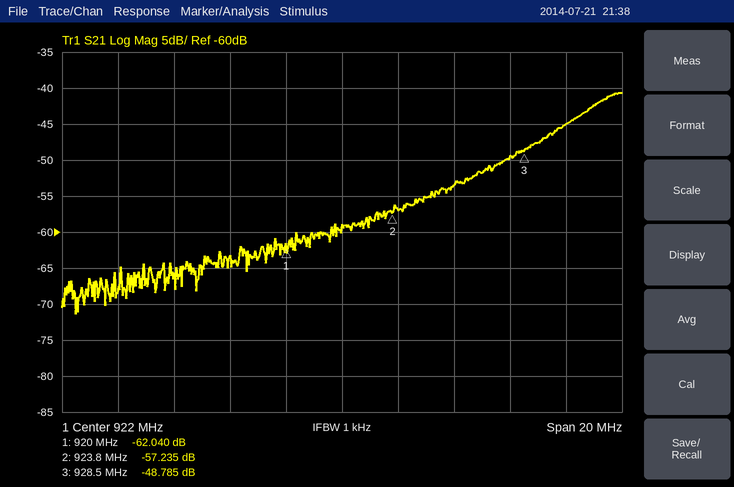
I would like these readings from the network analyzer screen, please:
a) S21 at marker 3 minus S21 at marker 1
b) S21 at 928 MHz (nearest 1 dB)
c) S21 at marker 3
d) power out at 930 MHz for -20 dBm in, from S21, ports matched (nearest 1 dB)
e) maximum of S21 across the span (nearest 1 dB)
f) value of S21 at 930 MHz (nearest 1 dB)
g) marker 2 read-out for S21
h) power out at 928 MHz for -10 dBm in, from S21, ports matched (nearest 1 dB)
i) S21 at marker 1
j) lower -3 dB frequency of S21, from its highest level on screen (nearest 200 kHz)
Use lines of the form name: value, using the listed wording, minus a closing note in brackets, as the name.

S21 at marker 3 minus S21 at marker 1: 13.255 dB
S21 at 928 MHz: -50 dB
S21 at marker 3: -48.785 dB
power out at 930 MHz for -20 dBm in, from S21, ports matched: -65 dBm
maximum of S21 across the span: -41 dB
value of S21 at 930 MHz: -45 dB
marker 2 read-out for S21: -57.235 dB
power out at 928 MHz for -10 dBm in, from S21, ports matched: -60 dBm
S21 at marker 1: -62.040 dB
lower -3 dB frequency of S21, from its highest level on screen: 930.6 MHz
